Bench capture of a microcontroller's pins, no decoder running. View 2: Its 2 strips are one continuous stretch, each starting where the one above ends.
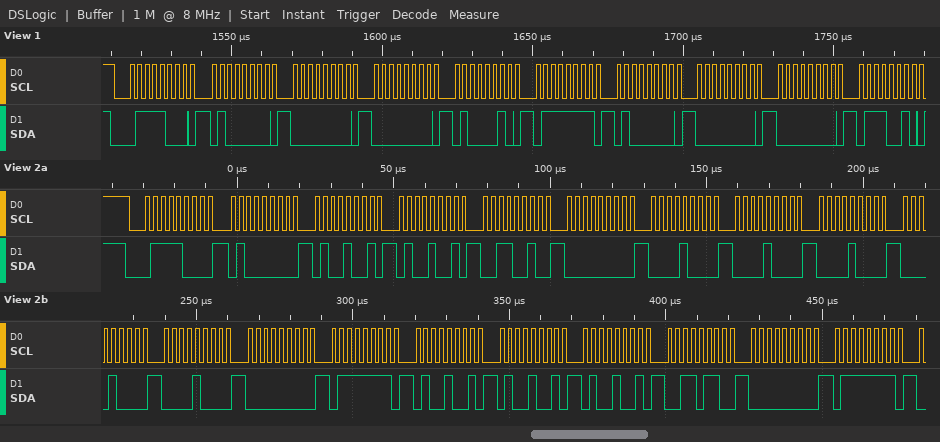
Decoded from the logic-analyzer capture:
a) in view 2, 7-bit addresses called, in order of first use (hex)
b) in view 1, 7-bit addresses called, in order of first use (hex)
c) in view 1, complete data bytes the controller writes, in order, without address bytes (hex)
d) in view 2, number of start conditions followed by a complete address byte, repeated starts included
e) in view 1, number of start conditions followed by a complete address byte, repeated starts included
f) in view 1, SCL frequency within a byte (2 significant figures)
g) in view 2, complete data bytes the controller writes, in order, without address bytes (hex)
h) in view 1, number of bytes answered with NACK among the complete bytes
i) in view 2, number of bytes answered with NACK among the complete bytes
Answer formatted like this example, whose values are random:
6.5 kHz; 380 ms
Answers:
0x3C; 0x3C; 40 00 00 42 7F 40 00 00 72; 1; 1; 400 kHz; 40 49 49 32 00 08 08 08 08 08 00 7F 49 49 49 36 00 7F; 0; 0
